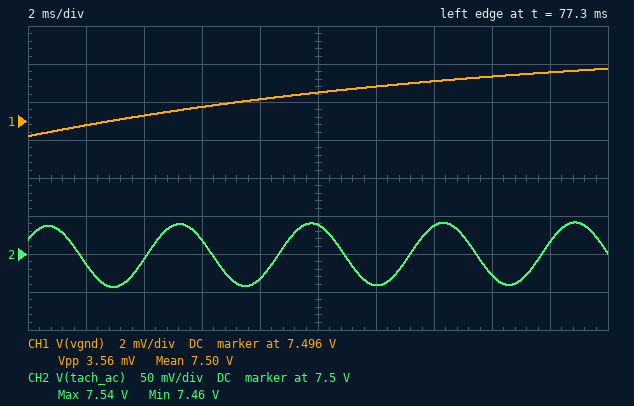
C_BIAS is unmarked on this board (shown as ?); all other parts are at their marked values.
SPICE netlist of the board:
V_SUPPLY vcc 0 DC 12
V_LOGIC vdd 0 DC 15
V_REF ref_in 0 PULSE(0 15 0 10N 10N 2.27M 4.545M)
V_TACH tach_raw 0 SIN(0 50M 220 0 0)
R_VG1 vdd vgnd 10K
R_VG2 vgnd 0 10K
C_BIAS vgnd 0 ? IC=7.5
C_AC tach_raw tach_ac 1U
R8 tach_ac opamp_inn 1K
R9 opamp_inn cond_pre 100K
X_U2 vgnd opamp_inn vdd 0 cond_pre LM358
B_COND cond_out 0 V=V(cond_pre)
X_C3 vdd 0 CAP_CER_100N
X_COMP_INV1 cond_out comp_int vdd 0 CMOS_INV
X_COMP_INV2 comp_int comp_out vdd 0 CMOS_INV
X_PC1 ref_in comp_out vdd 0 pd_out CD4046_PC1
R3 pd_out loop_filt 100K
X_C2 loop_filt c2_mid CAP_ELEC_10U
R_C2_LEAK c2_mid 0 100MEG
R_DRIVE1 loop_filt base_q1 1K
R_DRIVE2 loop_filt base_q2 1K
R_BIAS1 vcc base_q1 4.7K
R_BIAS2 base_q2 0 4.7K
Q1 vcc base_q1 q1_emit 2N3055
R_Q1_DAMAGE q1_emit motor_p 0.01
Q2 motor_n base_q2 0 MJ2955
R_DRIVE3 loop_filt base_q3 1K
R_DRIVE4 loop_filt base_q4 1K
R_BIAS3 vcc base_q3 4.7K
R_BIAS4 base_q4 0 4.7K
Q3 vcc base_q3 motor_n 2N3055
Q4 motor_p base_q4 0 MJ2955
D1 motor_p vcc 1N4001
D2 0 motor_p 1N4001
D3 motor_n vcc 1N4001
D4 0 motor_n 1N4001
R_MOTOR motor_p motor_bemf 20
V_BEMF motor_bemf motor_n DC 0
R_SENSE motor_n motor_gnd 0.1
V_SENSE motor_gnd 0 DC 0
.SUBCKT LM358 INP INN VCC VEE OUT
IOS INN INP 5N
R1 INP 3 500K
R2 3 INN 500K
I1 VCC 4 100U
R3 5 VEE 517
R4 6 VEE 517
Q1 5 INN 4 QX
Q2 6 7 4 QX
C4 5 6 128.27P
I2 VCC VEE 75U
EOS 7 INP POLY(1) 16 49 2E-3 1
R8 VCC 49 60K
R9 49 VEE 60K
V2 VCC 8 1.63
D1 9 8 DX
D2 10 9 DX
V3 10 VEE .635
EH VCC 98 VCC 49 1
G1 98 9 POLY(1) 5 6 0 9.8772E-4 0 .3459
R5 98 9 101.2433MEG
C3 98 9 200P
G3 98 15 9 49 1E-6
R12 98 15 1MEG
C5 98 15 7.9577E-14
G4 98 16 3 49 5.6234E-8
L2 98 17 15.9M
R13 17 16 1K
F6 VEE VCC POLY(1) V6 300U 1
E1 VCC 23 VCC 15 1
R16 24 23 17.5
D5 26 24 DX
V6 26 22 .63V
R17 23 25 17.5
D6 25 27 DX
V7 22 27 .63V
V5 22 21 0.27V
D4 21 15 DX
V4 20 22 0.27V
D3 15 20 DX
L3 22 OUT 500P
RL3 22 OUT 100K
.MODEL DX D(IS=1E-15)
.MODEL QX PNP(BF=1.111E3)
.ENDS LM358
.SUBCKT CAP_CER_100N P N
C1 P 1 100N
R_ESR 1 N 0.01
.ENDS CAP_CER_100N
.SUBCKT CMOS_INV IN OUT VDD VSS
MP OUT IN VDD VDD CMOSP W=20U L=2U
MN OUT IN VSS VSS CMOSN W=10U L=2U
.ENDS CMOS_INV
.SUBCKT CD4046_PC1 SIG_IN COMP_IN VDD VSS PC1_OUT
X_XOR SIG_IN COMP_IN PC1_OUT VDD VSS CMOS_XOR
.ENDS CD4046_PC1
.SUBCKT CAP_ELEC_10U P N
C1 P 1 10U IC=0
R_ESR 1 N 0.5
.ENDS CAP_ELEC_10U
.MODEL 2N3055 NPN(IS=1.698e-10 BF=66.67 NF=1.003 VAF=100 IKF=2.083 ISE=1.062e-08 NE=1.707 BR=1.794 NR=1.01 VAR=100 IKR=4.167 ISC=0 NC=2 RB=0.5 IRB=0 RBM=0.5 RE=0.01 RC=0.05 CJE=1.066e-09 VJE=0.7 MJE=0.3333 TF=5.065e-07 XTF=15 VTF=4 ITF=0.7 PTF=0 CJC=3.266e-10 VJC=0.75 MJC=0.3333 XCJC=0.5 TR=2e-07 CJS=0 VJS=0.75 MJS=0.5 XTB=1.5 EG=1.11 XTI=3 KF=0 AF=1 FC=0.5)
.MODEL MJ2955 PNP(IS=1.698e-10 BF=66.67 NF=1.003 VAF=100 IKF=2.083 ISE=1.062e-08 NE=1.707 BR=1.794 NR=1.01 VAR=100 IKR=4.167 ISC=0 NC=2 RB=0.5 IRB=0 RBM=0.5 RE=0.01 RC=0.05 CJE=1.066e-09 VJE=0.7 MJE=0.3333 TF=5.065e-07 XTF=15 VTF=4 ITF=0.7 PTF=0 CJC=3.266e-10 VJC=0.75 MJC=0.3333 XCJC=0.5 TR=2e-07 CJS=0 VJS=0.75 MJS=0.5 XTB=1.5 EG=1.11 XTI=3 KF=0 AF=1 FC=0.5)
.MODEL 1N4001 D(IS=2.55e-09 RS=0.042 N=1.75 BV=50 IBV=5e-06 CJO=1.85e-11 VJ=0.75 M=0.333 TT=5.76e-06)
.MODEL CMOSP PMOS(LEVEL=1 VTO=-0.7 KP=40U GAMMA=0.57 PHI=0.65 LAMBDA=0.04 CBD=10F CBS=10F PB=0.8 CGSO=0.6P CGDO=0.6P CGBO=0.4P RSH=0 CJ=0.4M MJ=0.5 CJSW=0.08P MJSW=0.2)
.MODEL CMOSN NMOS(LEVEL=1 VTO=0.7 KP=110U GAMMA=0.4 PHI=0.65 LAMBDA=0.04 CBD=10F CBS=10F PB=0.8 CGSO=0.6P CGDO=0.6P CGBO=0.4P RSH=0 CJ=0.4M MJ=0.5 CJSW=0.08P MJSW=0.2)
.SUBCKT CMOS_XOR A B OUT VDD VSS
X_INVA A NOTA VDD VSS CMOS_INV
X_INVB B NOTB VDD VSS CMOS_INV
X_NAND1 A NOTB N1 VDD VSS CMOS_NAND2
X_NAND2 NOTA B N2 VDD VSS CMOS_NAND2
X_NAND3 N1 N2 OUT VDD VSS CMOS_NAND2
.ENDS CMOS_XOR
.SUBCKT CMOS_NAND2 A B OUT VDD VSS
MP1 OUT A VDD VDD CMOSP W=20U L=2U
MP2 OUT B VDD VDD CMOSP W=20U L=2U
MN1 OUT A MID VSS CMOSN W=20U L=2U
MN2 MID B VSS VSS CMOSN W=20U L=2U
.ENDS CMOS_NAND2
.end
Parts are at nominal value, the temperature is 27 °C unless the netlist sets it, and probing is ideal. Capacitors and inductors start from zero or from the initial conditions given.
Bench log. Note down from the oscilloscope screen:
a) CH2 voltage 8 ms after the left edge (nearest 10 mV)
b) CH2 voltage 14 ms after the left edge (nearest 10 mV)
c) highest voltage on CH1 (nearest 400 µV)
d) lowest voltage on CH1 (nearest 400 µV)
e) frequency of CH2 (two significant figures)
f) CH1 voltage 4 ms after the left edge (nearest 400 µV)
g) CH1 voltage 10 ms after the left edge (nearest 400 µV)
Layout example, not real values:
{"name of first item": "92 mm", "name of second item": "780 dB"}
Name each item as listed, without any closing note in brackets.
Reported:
{"CH2 voltage 8 ms after the left edge": "7.47 V", "CH2 voltage 14 ms after the left edge": "7.54 V", "highest voltage on CH1": "7.4988 V", "lowest voltage on CH1": "7.4952 V", "frequency of CH2": "220 Hz", "CH1 voltage 4 ms after the left edge": "7.4964 V", "CH1 voltage 10 ms after the left edge": "7.4976 V"}
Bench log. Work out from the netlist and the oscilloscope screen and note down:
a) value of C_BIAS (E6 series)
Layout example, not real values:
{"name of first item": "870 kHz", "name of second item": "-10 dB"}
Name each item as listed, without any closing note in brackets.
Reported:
{"value of C_BIAS": "3.3 µF"}
